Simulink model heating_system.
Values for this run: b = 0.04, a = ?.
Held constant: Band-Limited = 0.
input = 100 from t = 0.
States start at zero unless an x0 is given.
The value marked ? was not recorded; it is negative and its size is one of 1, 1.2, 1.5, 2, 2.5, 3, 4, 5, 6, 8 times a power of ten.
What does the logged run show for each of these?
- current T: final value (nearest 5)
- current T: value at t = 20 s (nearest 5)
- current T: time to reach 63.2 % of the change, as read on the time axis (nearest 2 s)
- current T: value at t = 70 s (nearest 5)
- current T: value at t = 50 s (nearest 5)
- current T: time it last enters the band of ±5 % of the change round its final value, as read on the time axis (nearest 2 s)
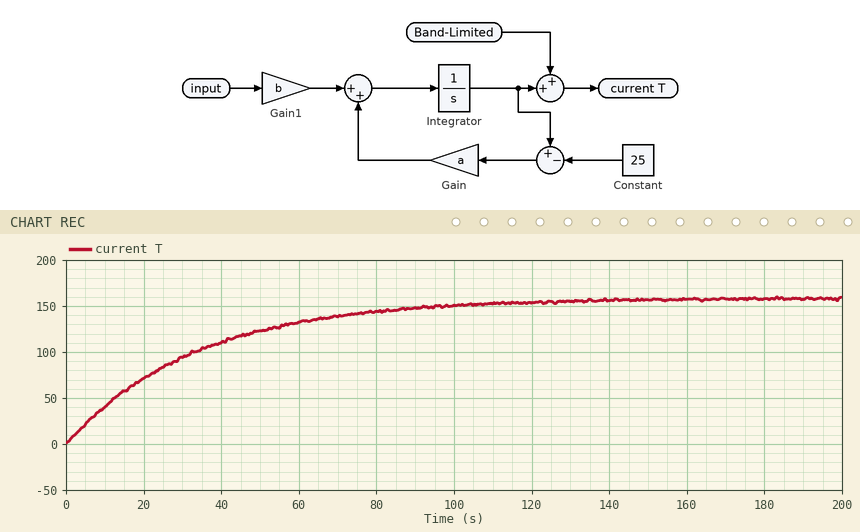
160
70
34 s
140
125
100 s
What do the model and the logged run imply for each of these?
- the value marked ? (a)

-0.03
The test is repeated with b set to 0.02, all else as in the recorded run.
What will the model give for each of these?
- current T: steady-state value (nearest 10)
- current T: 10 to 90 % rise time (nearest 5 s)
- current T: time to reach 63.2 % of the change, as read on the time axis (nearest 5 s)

90
75 s
35 s
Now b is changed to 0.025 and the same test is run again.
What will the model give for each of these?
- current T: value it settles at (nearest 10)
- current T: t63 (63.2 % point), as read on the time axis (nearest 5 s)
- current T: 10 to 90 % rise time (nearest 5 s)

110
35 s
75 s
